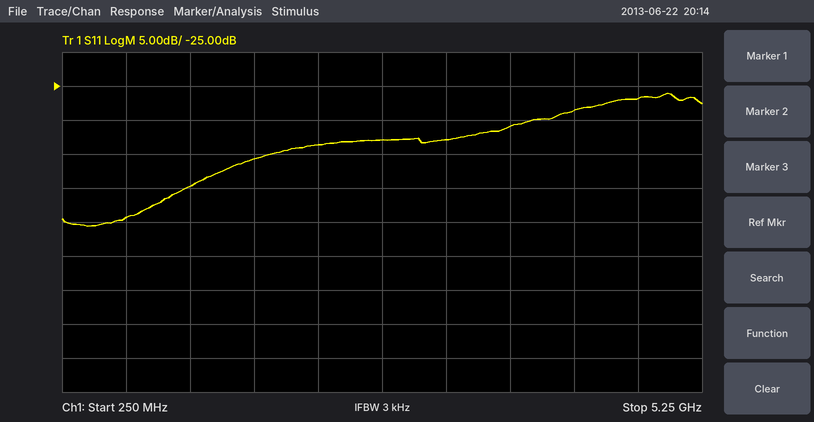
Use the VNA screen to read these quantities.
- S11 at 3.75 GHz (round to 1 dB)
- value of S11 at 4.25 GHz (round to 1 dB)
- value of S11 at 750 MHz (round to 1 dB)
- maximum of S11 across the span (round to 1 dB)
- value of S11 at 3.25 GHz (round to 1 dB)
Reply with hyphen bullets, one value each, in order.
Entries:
- -31 dB
- -29 dB
- -44 dB
- -26 dB
- -33 dB
